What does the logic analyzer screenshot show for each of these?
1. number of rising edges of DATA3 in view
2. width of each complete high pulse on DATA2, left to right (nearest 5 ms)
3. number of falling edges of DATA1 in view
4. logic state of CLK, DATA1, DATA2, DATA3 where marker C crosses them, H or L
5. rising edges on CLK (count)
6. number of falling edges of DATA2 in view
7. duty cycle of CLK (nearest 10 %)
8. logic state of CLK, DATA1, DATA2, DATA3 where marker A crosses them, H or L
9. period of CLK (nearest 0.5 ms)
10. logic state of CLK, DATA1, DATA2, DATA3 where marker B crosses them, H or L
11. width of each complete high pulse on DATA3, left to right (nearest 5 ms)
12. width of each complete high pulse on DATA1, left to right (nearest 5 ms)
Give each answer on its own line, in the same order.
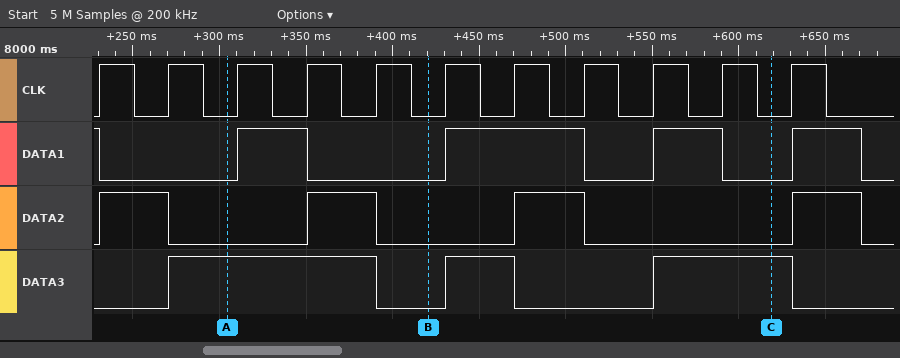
3
40 ms, 40 ms, 40 ms, 40 ms
5
CLK=L, DATA1=L, DATA2=L, DATA3=H
11
4
50 %
CLK=L, DATA1=L, DATA2=L, DATA3=H
40 ms
CLK=L, DATA1=L, DATA2=L, DATA3=L
120 ms, 40 ms, 80 ms
40 ms, 80 ms, 40 ms, 40 ms
